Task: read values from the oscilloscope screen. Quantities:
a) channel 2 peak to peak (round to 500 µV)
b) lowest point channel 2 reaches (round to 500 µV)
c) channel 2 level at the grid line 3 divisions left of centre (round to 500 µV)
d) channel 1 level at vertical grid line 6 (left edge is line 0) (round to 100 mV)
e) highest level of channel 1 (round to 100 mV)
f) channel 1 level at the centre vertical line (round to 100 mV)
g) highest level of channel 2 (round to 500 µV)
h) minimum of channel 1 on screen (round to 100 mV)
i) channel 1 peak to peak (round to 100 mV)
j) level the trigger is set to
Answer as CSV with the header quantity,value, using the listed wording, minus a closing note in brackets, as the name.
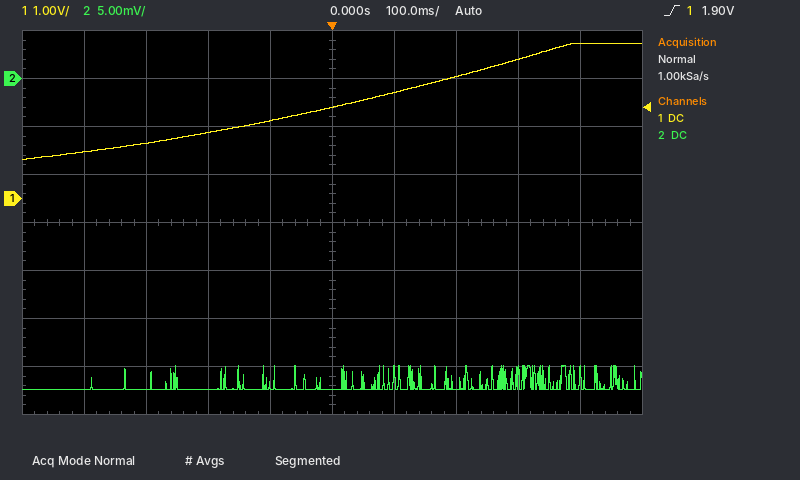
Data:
quantity,value
channel 2 peak to peak,2.5 mV
lowest point channel 2 reaches,-32.5 mV
channel 2 level at the grid line 3 divisions left of centre,-32.5 mV
channel 1 level at vertical grid line 6 (left edge is line 0),2.2 V
highest level of channel 1,3.2 V
channel 1 level at the centre vertical line,1.9 V
highest level of channel 2,-30.0 mV
minimum of channel 1 on screen,800 mV
channel 1 peak to peak,2.4 V
level the trigger is set to,1.90 V
